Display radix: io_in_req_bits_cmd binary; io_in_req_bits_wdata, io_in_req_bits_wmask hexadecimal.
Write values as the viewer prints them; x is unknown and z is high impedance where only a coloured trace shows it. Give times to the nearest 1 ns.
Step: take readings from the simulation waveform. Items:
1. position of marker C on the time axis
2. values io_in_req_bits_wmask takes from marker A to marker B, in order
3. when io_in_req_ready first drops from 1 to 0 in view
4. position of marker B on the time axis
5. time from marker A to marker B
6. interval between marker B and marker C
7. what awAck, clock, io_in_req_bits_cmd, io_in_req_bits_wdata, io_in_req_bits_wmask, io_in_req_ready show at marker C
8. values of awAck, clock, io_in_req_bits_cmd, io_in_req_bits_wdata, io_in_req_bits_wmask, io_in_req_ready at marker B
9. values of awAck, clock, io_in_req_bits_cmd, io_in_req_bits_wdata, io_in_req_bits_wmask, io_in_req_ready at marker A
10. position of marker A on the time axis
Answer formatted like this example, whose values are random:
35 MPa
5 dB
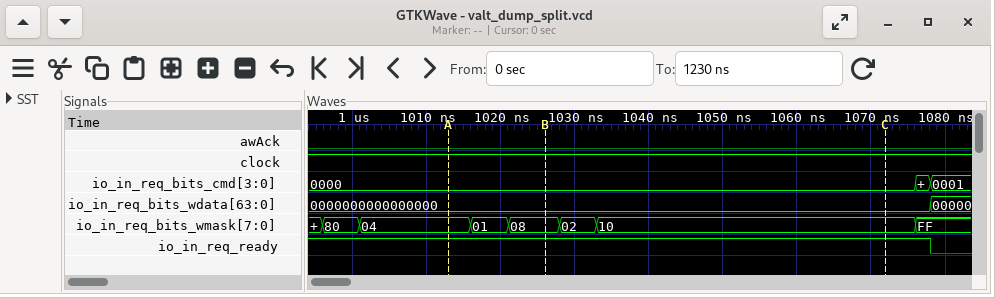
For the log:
1072 ns
04, 01, 08
1078 ns
1026 ns
13 ns
46 ns
awAck=0, clock=1, io_in_req_bits_cmd=0000, io_in_req_bits_wdata=0000000000000000, io_in_req_bits_wmask=10, io_in_req_ready=1
awAck=0, clock=1, io_in_req_bits_cmd=0000, io_in_req_bits_wdata=0000000000000000, io_in_req_bits_wmask=08, io_in_req_ready=1
awAck=0, clock=1, io_in_req_bits_cmd=0000, io_in_req_bits_wdata=0000000000000000, io_in_req_bits_wmask=04, io_in_req_ready=1
1013 ns
